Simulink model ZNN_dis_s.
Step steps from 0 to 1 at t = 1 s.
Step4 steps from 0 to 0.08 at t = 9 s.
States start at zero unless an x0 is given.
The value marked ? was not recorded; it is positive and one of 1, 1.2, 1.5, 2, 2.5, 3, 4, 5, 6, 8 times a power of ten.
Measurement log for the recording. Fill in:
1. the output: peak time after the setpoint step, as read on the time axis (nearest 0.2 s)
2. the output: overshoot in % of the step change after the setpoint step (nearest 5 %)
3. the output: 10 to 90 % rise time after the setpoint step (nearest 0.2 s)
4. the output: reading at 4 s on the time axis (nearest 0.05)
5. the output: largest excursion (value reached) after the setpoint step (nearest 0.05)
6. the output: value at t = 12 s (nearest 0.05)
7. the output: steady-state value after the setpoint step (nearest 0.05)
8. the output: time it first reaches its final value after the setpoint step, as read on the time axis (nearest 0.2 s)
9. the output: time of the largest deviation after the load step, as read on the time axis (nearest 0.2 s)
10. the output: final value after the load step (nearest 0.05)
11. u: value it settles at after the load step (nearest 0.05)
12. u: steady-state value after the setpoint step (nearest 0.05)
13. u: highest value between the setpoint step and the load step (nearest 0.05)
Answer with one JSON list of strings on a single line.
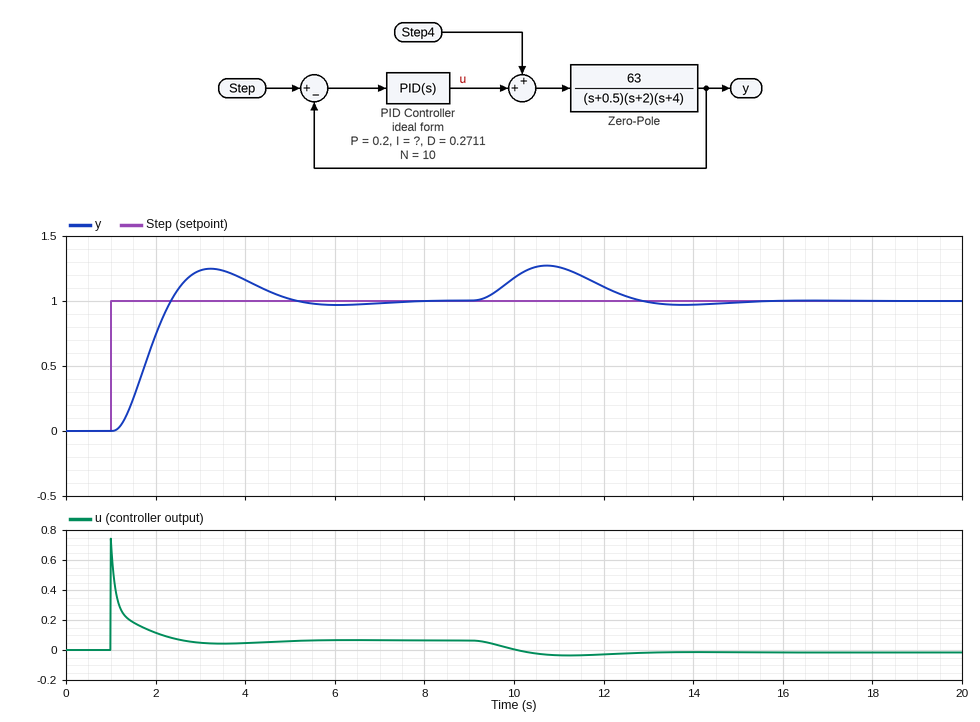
["3.2 s", "25 %", "0.8 s", "1.15", "1.25", "1.10", "1.00", "2.4 s", "10.8 s", "1.00", "0.00", "0.05", "0.75"]
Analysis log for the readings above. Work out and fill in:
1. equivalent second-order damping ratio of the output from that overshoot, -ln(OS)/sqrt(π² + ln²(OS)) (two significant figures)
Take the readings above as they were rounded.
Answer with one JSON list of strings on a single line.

["0.40"]
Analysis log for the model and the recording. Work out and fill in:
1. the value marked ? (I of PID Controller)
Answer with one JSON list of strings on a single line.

["0.8"]
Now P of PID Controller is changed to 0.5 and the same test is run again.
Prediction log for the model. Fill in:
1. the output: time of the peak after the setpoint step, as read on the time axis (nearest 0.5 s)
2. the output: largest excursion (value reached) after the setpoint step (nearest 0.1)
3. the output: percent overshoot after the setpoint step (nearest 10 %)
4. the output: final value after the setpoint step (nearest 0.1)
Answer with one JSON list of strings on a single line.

["2.0 s", "1.4", "40 %", "1.0"]
